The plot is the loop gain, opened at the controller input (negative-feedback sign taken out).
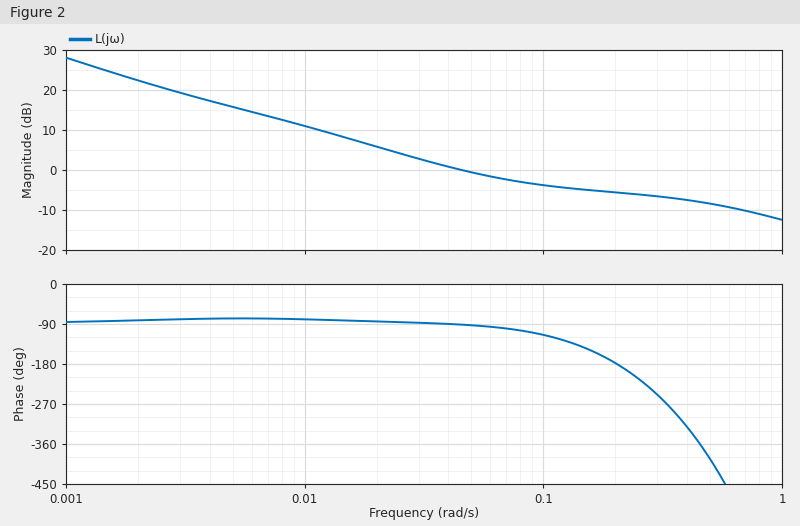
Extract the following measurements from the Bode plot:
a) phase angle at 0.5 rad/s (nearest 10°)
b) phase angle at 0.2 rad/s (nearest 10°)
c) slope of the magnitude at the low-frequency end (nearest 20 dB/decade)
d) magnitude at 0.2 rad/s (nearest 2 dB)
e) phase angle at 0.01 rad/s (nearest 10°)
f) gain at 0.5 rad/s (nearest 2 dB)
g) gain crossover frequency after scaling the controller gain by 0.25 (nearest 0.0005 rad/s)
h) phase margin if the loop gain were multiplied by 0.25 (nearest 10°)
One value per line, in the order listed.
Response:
-390°
-180°
-20 dB/decade
-6 dB
-80°
-8 dB
0.0085 rad/s
100°
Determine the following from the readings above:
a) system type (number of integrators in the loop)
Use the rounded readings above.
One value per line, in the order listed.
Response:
1
